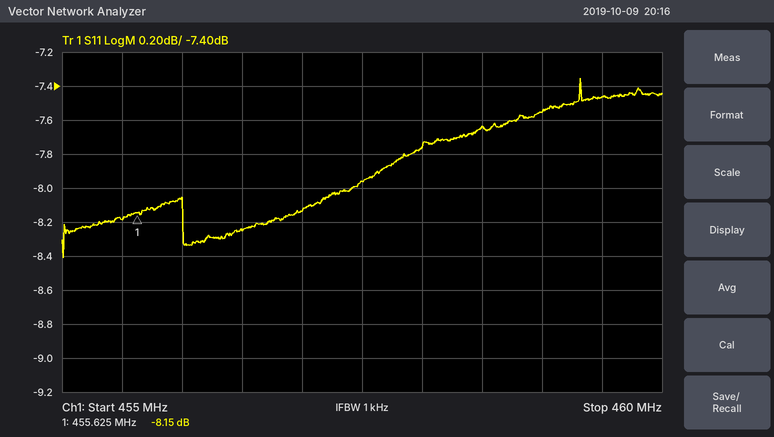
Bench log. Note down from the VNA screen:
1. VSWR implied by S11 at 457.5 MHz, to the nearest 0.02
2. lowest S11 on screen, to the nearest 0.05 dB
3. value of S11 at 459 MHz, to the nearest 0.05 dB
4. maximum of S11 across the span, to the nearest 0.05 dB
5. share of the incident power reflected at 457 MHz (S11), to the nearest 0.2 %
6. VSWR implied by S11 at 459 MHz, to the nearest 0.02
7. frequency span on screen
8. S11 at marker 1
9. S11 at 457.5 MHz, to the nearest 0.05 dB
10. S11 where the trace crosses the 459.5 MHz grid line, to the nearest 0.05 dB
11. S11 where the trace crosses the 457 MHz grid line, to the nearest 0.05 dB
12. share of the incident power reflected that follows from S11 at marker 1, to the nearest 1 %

2.34
-8.40 dB
-7.55 dB
-7.35 dB
15.4 %
2.44
5 MHz
-8.15 dB
-7.95 dB
-7.45 dB
-8.15 dB
15 %
